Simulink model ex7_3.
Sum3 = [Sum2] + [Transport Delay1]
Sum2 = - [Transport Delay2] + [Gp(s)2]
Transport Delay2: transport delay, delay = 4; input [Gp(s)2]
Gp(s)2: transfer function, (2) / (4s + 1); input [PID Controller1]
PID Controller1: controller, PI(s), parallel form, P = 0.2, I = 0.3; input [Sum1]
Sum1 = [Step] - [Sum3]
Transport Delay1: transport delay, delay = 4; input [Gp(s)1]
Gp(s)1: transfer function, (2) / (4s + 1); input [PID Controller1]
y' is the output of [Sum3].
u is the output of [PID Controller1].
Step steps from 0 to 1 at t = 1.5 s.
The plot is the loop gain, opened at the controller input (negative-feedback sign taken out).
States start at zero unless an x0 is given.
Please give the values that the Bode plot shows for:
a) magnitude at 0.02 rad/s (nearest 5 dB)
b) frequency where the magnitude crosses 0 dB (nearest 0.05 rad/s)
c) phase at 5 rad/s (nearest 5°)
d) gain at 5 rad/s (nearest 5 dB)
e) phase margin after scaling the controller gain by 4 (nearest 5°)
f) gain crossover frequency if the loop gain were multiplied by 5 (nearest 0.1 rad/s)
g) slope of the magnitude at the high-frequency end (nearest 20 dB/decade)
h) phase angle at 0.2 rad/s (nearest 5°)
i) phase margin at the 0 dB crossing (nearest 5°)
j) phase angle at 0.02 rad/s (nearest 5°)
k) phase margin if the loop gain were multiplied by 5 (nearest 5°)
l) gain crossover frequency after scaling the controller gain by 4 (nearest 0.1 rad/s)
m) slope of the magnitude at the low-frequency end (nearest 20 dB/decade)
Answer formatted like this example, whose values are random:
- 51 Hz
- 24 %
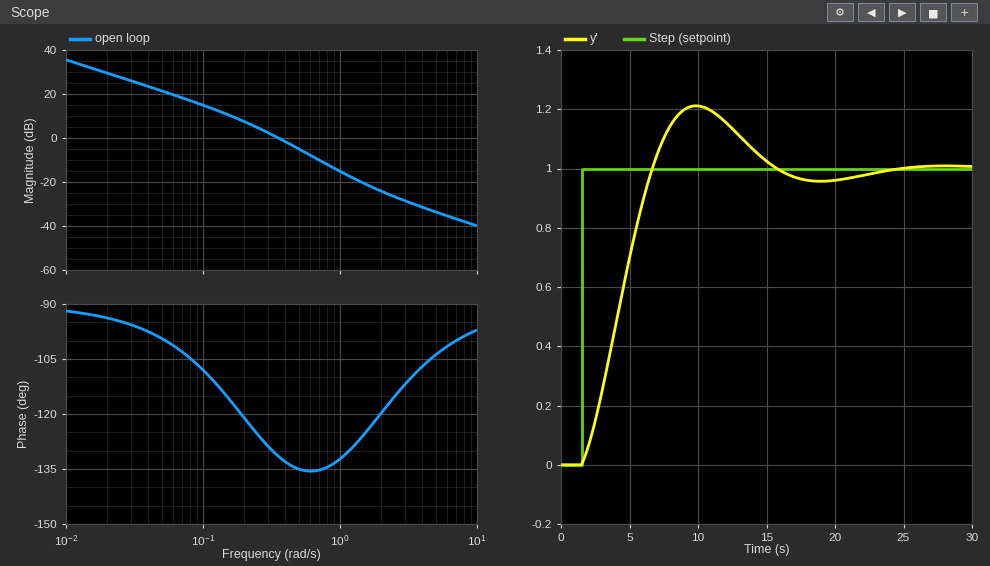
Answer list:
- 30 dB
- 0.35 rad/s
- -105°
- -35 dB
- 45°
- 0.9 rad/s
- -20 dB/decade
- -120°
- 50°
- -95°
- 45°
- 0.8 rad/s
- -20 dB/decade
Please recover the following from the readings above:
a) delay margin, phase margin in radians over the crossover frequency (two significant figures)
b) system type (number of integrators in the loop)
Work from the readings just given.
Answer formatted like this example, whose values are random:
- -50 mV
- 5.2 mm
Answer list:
- 2.5 s
- 1
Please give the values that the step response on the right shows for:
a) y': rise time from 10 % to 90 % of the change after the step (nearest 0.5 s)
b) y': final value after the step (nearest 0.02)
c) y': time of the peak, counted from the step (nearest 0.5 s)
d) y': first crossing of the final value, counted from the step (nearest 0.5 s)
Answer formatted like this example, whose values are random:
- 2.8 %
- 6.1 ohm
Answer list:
- 4.0 s
- 1.00
- 8.5 s
- 5.0 s
